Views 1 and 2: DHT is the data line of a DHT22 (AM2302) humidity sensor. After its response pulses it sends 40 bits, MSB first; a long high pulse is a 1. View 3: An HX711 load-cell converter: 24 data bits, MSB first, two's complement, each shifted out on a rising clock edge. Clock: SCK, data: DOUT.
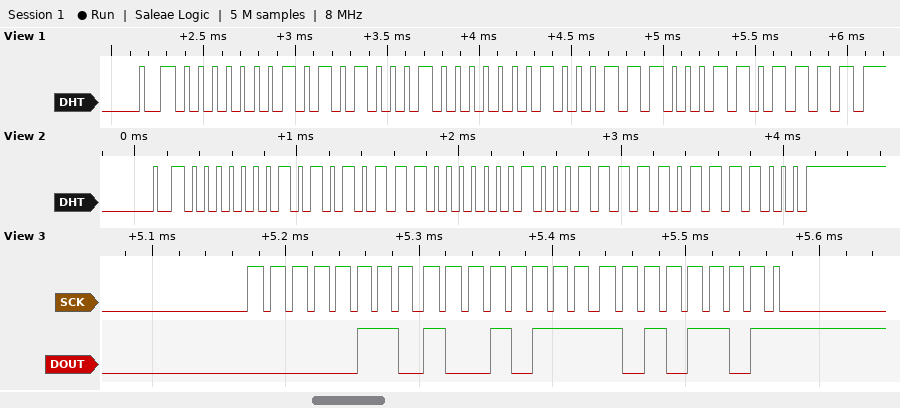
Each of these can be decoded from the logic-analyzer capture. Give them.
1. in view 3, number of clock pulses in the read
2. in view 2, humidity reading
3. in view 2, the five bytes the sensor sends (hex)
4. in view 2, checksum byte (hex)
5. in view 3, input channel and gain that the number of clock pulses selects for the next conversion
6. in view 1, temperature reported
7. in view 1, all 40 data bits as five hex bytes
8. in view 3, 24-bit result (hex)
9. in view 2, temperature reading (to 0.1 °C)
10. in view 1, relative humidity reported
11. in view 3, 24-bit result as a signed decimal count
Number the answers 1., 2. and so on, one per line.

1. 25
2. 34.3 %
3. 01 57 01 1F 78
4. 0x78
5. channel A, gain 128
6. 28.4 °C
7. 01 51 01 1C 6F
8. 0x0697AD
9. 28.7 °C
10. 33.7 %
11. 432045
